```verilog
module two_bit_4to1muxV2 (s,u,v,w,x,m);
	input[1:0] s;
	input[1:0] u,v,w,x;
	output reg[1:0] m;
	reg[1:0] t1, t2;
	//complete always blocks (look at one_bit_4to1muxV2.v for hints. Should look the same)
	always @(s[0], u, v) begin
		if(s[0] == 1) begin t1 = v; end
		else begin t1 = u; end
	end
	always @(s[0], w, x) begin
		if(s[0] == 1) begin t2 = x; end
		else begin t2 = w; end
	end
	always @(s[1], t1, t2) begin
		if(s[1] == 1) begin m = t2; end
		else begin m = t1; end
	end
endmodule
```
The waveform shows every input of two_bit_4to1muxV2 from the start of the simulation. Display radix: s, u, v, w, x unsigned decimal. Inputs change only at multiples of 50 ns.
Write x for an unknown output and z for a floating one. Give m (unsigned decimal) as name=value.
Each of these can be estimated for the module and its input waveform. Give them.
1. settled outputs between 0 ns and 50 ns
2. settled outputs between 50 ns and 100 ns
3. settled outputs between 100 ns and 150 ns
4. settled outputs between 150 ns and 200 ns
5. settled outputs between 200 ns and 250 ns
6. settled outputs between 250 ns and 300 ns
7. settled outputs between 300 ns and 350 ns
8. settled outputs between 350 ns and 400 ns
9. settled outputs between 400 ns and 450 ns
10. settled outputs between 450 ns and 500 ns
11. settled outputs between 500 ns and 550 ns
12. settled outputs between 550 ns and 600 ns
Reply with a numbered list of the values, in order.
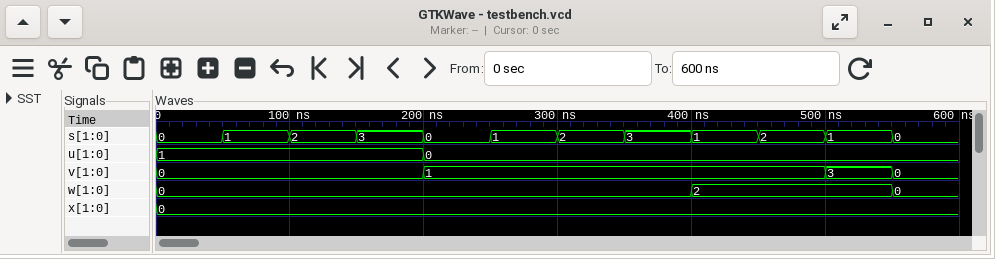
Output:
1. m=1
2. m=0
3. m=0
4. m=0
5. m=0
6. m=1
7. m=0
8. m=0
9. m=1
10. m=2
11. m=3
12. m=0
